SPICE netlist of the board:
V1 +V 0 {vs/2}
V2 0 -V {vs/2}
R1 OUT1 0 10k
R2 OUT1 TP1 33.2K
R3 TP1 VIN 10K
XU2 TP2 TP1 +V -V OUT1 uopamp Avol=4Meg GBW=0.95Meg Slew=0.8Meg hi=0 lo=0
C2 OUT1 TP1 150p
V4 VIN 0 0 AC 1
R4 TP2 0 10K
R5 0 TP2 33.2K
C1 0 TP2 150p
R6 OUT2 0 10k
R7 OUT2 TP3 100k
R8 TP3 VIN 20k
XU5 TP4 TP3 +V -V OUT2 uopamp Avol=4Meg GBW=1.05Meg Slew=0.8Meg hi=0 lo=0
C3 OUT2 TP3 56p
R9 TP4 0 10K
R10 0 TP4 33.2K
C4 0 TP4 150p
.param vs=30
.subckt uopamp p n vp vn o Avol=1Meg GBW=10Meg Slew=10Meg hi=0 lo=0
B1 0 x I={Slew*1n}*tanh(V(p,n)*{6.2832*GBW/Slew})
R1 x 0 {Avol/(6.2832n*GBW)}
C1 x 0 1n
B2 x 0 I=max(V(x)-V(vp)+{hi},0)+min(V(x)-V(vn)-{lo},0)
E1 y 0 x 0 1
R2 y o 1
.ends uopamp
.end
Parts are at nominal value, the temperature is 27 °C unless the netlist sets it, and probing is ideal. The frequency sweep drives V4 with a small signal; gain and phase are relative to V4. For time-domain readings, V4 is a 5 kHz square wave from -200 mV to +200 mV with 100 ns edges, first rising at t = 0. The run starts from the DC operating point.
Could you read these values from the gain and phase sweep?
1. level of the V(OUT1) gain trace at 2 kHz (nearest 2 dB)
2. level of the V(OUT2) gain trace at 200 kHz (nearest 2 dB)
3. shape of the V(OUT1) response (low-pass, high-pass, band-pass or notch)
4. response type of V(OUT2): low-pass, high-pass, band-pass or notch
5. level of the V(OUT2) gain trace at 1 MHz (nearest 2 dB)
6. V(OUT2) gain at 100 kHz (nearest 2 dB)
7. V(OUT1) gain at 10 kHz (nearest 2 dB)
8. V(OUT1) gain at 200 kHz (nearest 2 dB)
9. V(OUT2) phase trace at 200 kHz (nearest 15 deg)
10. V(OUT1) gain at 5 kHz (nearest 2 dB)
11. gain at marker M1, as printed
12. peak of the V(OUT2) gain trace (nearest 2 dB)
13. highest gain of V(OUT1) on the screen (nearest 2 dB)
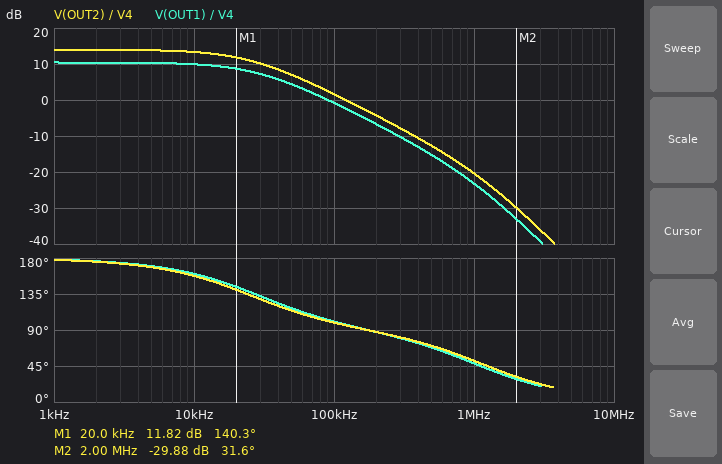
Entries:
10 dB
-4 dB
low-pass
low-pass
-20 dB
2 dB
10 dB
-6 dB
90 deg
10 dB
11.82 dB
14 dB
10 dB
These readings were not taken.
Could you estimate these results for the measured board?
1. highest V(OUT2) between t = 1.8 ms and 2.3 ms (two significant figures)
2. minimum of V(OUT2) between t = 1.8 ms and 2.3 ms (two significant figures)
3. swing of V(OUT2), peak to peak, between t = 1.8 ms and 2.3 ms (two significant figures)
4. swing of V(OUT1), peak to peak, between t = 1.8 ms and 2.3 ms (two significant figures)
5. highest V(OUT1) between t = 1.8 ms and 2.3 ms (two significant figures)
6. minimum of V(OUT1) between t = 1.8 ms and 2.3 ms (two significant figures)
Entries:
1.0 V
-1.0 V
2.0 V
1.3 V
660 mV
-660 mV
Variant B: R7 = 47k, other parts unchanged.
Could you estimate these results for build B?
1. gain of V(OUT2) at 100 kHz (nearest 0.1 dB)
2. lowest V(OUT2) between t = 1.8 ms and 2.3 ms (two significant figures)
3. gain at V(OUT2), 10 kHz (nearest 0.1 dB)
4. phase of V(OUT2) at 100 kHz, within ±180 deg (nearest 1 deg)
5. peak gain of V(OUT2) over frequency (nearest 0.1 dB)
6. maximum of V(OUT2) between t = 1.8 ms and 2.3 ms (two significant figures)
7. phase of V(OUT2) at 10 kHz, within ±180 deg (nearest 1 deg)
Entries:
0.8 dB
-470 mV
7.3 dB
113 deg
7.4 dB
470 mV
169 deg
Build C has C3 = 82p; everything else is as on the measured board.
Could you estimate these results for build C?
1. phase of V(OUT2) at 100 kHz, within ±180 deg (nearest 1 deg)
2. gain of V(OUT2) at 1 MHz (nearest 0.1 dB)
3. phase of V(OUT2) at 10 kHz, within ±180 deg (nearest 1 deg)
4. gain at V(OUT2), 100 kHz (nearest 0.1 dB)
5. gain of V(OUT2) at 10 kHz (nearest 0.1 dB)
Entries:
95 deg
-23.5 dB
150 deg
-1.2 dB
12.8 dB
